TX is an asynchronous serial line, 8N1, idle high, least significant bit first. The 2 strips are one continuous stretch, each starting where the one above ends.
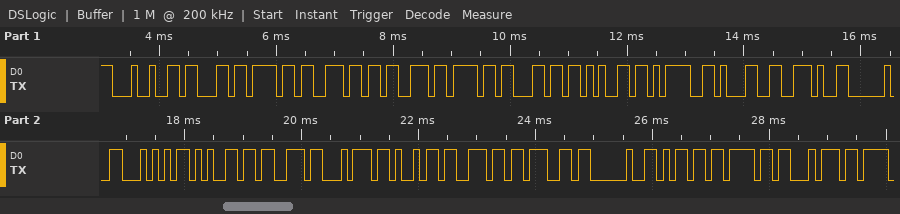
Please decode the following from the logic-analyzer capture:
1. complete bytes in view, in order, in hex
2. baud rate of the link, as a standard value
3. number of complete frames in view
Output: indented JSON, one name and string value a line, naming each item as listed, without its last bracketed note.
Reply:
{
  "complete bytes in view, in order, in hex": "24 63 6F 6E 73 6F 6C 65 3D 31 2E 20 54 65 73 74 69 6E 67 20 6D 6F 74",
  "baud rate of the link, as a standard value": "9600 baud",
  "number of complete frames in view": "23"
}
